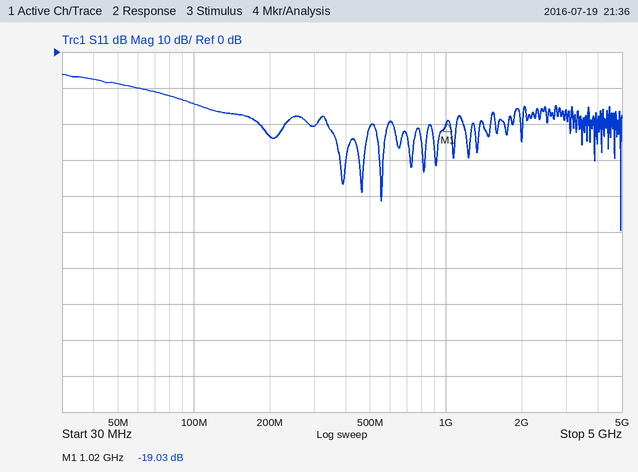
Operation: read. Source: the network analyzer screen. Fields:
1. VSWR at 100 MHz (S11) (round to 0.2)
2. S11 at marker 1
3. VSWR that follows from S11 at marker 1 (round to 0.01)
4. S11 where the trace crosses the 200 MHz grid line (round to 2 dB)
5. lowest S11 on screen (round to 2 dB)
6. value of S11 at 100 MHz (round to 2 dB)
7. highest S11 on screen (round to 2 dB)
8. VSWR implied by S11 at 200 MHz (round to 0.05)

1.4
-19.03 dB
1.25
-24 dB
-50 dB
-14 dB
-6 dB
1.15
